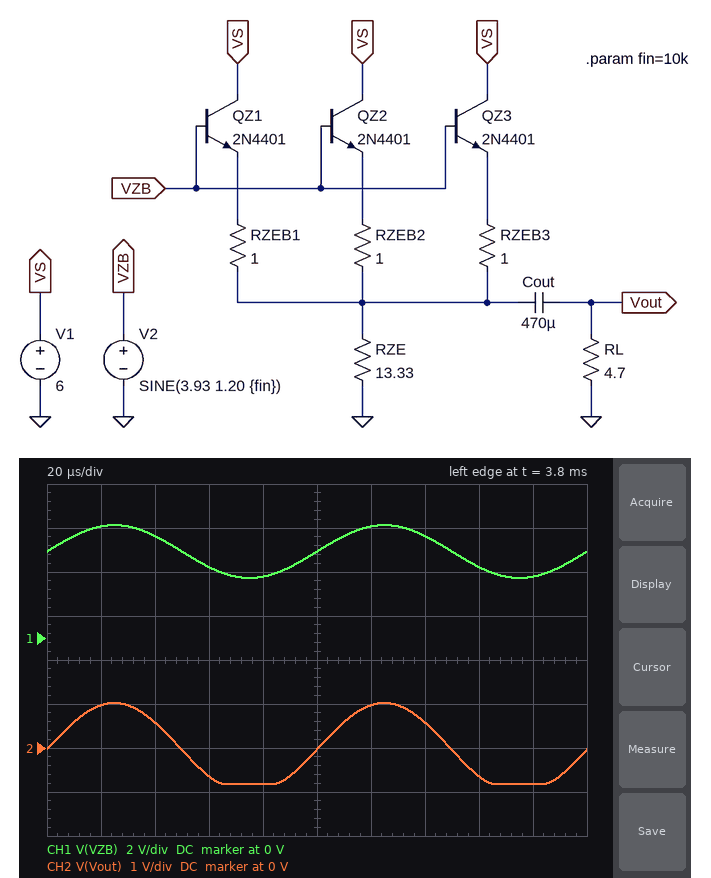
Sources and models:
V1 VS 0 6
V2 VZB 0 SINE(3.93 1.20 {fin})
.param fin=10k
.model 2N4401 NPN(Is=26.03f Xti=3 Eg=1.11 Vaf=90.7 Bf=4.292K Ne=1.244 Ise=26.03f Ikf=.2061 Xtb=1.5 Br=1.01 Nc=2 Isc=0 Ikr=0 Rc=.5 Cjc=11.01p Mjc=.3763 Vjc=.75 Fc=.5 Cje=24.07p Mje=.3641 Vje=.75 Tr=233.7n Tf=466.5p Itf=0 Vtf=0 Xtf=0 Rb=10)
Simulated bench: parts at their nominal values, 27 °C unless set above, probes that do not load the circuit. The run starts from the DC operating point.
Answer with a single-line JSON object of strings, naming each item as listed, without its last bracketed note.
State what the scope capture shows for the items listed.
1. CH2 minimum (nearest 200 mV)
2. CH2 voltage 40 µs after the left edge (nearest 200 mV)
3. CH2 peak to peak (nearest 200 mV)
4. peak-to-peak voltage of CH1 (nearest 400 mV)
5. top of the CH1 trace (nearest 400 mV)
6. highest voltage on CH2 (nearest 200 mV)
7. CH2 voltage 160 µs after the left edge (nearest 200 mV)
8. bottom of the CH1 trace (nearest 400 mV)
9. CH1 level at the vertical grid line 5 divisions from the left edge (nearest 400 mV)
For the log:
{"CH2 minimum": "-800 mV", "CH2 voltage 40 µs after the left edge": "600 mV", "CH2 peak to peak": "1.8 V", "peak-to-peak voltage of CH1": "2.4 V", "top of the CH1 trace": "5.2 V", "highest voltage on CH2": "1.0 V", "CH2 voltage 160 µs after the left edge": "-600 mV", "bottom of the CH1 trace": "2.8 V", "CH1 level at the vertical grid line 5 divisions from the left edge": "4.0 V"}
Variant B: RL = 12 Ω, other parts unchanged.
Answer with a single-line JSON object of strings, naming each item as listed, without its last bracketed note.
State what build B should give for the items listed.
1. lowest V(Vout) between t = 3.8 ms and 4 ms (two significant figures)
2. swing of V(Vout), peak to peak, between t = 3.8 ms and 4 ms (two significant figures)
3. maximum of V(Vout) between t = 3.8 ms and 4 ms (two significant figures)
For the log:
{"lowest V(Vout) between t = 3.8 ms and 4 ms": "-1.1 V", "swing of V(Vout), peak to peak, between t = 3.8 ms and 4 ms": "2.2 V", "maximum of V(Vout) between t = 3.8 ms and 4 ms": "1.1 V"}
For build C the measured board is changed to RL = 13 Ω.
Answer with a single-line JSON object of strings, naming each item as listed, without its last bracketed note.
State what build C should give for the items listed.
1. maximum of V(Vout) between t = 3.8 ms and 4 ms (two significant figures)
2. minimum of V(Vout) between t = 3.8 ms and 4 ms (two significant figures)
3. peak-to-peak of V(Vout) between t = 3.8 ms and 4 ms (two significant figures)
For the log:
{"maximum of V(Vout) between t = 3.8 ms and 4 ms": "1.1 V", "minimum of V(Vout) between t = 3.8 ms and 4 ms": "-1.1 V", "peak-to-peak of V(Vout) between t = 3.8 ms and 4 ms": "2.2 V"}
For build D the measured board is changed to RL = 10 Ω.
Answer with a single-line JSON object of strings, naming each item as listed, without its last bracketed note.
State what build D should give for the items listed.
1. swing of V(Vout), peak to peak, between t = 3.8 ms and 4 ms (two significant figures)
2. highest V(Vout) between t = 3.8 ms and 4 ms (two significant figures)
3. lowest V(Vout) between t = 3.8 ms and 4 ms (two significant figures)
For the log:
{"swing of V(Vout), peak to peak, between t = 3.8 ms and 4 ms": "2.2 V", "highest V(Vout) between t = 3.8 ms and 4 ms": "1.1 V", "lowest V(Vout) between t = 3.8 ms and 4 ms": "-1.1 V"}
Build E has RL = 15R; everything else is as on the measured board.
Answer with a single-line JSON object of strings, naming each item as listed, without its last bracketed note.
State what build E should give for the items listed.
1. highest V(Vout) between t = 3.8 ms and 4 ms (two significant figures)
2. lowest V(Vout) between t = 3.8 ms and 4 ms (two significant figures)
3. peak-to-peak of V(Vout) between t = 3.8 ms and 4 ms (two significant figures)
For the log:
{"highest V(Vout) between t = 3.8 ms and 4 ms": "1.1 V", "lowest V(Vout) between t = 3.8 ms and 4 ms": "-1.1 V", "peak-to-peak of V(Vout) between t = 3.8 ms and 4 ms": "2.2 V"}
